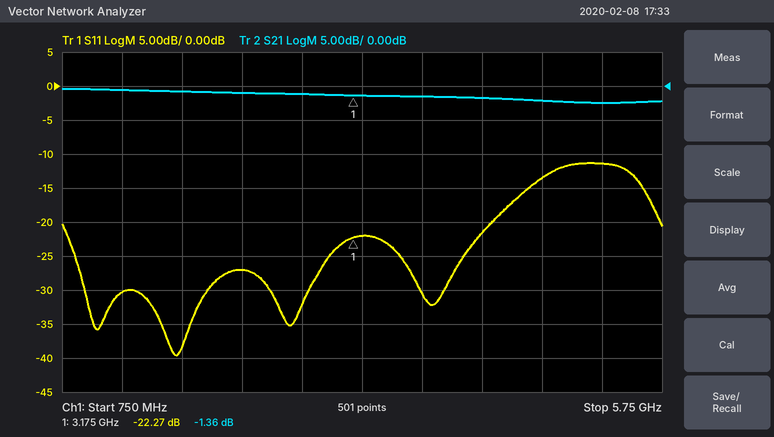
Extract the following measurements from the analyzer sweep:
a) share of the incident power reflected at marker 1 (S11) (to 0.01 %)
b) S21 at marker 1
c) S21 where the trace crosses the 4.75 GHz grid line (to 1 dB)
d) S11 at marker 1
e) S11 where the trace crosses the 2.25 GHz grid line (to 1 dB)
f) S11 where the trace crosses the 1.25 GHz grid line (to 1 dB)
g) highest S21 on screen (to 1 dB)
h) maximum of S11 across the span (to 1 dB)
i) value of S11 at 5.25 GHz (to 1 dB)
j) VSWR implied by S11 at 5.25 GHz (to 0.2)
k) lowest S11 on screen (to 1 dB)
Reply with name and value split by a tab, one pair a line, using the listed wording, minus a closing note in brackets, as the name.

share of the incident power reflected at marker 1 (S11)	0.59 %
S21 at marker 1	-1.36 dB
S21 where the trace crosses the 4.75 GHz grid line	-2 dB
S11 at marker 1	-22.27 dB
S11 where the trace crosses the 2.25 GHz grid line	-27 dB
S11 where the trace crosses the 1.25 GHz grid line	-30 dB
highest S21 on screen	0 dB
maximum of S11 across the span	-11 dB
value of S11 at 5.25 GHz	-11 dB
VSWR implied by S11 at 5.25 GHz	1.8
lowest S11 on screen	-40 dB
